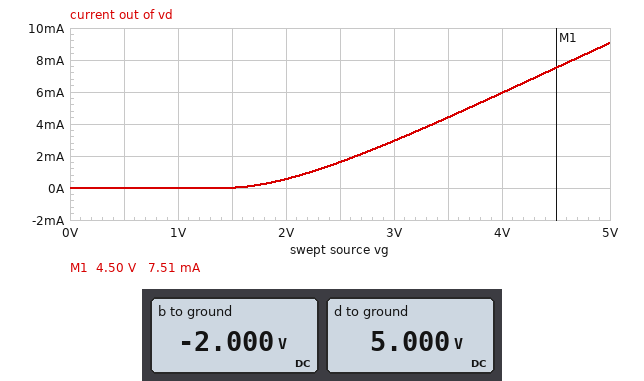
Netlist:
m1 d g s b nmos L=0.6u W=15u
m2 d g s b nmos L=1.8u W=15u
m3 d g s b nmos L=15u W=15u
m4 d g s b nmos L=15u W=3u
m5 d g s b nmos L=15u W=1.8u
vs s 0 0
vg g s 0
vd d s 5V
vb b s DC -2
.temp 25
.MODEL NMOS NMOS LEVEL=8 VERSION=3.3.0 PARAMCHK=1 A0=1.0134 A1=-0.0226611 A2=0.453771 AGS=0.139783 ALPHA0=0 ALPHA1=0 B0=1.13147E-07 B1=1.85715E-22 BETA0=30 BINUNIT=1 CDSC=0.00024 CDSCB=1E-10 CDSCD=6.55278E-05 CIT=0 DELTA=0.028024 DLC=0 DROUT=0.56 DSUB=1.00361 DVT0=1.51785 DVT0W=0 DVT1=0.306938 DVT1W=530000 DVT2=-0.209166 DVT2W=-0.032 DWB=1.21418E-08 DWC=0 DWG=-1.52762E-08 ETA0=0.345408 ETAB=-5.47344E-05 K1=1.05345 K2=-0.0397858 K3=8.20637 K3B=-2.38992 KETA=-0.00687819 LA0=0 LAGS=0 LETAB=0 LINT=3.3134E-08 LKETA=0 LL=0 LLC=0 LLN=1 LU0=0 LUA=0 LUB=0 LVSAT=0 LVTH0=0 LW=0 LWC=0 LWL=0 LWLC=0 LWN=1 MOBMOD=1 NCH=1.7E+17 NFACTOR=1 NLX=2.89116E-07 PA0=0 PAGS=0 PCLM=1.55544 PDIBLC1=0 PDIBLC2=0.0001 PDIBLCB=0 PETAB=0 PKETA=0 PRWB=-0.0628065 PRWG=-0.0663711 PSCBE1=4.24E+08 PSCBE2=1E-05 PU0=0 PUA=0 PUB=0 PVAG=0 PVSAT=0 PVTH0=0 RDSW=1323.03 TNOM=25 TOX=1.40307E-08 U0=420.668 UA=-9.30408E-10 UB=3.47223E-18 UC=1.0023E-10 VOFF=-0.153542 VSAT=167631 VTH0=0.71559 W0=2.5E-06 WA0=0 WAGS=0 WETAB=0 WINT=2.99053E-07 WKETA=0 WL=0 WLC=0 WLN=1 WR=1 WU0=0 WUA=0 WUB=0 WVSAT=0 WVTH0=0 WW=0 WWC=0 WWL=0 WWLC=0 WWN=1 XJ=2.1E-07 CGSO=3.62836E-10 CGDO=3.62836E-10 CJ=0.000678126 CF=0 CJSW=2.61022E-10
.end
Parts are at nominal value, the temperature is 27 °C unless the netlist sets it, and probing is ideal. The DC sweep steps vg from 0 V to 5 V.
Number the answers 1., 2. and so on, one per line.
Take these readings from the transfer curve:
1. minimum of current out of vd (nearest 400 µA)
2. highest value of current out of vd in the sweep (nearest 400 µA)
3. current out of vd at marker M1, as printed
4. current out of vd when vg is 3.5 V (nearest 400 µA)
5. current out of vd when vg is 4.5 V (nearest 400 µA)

1. 0 A
2. 9.2 mA
3. 7.51 mA
4. 4.4 mA
5. 7.6 mA
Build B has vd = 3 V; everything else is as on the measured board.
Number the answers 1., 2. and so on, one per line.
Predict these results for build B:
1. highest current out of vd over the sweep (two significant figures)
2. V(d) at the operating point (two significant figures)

1. 8.9 mA
2. 3.0 V
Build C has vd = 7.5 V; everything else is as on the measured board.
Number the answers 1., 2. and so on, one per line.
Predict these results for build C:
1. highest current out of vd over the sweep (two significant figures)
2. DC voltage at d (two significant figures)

1. 10 mA
2. 7.5 V
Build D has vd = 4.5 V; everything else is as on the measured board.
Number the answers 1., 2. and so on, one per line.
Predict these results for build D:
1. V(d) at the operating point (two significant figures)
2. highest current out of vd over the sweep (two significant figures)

1. 4.5 V
2. 9.0 mA
